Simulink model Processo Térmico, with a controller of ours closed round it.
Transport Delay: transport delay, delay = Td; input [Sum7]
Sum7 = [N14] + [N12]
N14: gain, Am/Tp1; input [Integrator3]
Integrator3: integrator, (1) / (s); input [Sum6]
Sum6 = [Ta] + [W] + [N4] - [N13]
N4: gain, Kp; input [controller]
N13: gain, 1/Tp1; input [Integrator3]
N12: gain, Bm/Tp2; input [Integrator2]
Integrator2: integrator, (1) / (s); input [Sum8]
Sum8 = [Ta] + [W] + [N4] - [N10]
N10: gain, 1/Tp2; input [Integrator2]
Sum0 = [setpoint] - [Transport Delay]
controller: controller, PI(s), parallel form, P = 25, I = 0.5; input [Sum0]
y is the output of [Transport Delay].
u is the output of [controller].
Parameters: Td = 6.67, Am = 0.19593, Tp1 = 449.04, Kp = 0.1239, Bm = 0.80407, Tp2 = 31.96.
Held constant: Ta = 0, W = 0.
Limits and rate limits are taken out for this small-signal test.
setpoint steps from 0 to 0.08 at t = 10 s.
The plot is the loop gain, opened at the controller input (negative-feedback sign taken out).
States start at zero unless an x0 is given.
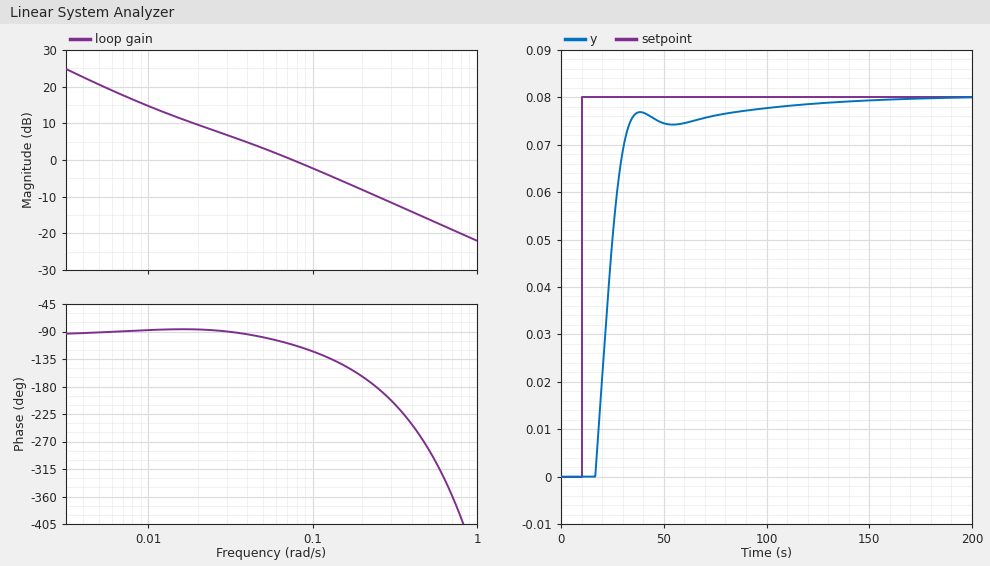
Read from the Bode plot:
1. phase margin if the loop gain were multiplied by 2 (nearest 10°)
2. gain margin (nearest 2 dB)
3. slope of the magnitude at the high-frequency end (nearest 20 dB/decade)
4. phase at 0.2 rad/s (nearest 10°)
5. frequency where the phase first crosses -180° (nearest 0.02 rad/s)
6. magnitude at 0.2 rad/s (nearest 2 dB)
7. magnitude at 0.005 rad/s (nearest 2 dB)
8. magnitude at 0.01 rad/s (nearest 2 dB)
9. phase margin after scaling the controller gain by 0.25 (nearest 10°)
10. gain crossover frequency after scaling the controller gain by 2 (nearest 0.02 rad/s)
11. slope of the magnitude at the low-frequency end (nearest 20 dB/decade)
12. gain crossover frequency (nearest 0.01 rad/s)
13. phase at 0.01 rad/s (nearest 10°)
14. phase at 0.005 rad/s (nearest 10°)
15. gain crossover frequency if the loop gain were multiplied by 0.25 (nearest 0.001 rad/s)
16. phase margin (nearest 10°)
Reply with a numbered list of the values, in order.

1. 30°
2. 10 dB
3. -20 dB/decade
4. -160°
5. 0.24 rad/s
6. -8 dB
7. 20 dB
8. 14 dB
9. 90°
10. 0.16 rad/s
11. -20 dB/decade
12. 0.08 rad/s
13. -90°
14. -90°
15. 0.014 rad/s
16. 70°
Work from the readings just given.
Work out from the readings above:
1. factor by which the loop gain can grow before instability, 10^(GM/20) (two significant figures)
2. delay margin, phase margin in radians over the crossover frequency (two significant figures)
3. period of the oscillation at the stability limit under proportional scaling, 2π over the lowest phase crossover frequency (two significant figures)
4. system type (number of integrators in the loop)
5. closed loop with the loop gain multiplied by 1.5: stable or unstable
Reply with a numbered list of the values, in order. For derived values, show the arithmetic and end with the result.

1. 10^(10 / 20) = 3.2
2. 70 × π / 180 / 0.08 = 15 s
3. 2π / 0.24 = 26 s
4. 1
5. stable
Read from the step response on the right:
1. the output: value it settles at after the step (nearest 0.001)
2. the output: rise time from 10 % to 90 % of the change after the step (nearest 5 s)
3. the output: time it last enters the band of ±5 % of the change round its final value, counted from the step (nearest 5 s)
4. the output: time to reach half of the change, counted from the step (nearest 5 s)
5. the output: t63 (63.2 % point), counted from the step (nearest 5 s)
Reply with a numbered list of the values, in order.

1. 0.080
2. 15 s
3. 65 s
4. 15 s
5. 15 s
